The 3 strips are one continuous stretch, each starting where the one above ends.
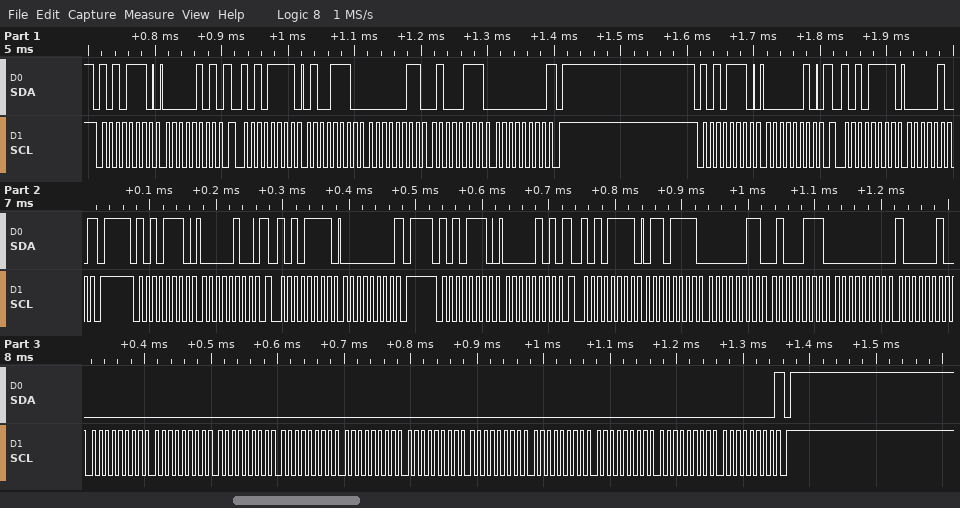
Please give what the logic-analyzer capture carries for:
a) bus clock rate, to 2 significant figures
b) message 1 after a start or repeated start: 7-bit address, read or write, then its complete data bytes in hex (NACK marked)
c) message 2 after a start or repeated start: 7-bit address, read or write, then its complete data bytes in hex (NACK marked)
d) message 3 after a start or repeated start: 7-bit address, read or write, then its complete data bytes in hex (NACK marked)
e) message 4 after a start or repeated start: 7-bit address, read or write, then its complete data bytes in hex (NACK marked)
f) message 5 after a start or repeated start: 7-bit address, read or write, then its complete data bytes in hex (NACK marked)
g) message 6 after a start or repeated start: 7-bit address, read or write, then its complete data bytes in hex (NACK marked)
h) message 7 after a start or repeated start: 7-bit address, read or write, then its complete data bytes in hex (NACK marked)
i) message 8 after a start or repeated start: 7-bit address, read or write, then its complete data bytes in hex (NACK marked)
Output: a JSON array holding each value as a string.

["100 kHz", "0x57 write: 05", "0x57 read: 4E 03 47 00 NACK", "0x57 write: 02", "0x57 read: 04 NACK", "0x57 write: 04", "0x57 read: 00 NACK", "0x57 write: 05", "0x57 read: 6F 03 47 00 82 00 00 00 00 00 00 00 00 00 00 00 NACK"]
